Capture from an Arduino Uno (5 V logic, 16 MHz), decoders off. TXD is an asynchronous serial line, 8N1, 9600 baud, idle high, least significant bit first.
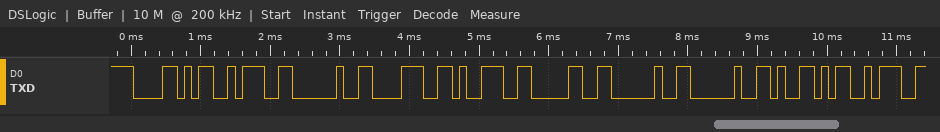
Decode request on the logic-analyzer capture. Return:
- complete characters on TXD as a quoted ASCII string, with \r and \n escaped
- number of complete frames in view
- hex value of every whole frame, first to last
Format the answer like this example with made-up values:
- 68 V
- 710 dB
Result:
- "X: 890  Y:"
- 10
- 0x58 0x3A 0x20 0x38 0x39 0x30 0x20 0x20 0x59 0x3A
